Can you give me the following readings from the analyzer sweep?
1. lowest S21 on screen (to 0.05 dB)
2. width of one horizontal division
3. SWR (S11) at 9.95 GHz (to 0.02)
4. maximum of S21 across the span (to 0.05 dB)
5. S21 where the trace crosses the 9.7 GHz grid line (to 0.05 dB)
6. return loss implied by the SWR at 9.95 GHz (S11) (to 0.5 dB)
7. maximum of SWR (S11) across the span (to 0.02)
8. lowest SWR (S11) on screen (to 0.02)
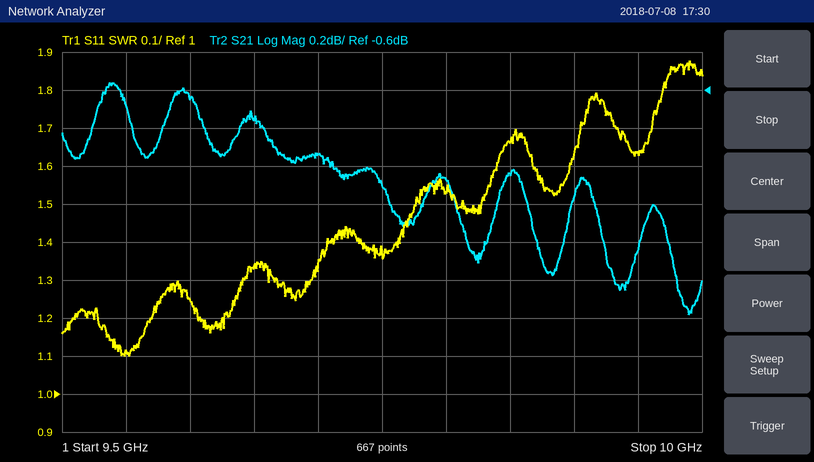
-1.80 dB
50 MHz
1.64
-0.55 dB
-0.95 dB
12.5 dB
1.88
1.10
